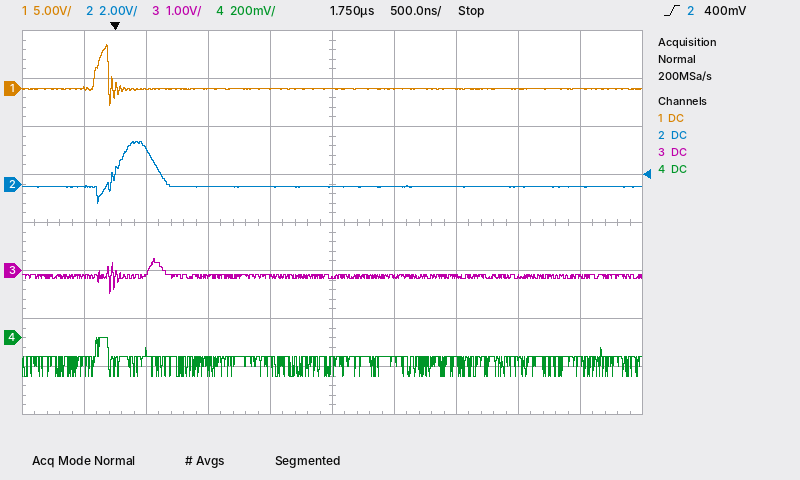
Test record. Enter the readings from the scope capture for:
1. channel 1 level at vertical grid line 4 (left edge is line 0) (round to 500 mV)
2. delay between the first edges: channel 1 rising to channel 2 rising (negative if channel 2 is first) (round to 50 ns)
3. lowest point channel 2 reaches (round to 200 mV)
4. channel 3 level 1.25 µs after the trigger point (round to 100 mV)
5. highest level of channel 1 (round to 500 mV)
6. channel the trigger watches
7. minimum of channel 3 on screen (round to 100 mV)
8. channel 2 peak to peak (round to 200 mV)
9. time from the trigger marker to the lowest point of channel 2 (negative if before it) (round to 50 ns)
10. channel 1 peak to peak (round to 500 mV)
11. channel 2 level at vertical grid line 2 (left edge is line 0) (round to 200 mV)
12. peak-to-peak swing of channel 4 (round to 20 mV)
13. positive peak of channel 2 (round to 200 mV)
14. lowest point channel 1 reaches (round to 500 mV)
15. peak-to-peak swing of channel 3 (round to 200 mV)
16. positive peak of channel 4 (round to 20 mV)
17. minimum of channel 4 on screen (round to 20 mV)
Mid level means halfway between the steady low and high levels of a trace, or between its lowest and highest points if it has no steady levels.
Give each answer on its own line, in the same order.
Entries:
0.0 V
+150 ns
-800 mV
-100 mV
4.5 V
channel 2
-500 mV
2.6 V
-150 ns
6.5 V
1.4 V
160 mV
1.8 V
-2.0 V
800 mV
0 mV
-160 mV
